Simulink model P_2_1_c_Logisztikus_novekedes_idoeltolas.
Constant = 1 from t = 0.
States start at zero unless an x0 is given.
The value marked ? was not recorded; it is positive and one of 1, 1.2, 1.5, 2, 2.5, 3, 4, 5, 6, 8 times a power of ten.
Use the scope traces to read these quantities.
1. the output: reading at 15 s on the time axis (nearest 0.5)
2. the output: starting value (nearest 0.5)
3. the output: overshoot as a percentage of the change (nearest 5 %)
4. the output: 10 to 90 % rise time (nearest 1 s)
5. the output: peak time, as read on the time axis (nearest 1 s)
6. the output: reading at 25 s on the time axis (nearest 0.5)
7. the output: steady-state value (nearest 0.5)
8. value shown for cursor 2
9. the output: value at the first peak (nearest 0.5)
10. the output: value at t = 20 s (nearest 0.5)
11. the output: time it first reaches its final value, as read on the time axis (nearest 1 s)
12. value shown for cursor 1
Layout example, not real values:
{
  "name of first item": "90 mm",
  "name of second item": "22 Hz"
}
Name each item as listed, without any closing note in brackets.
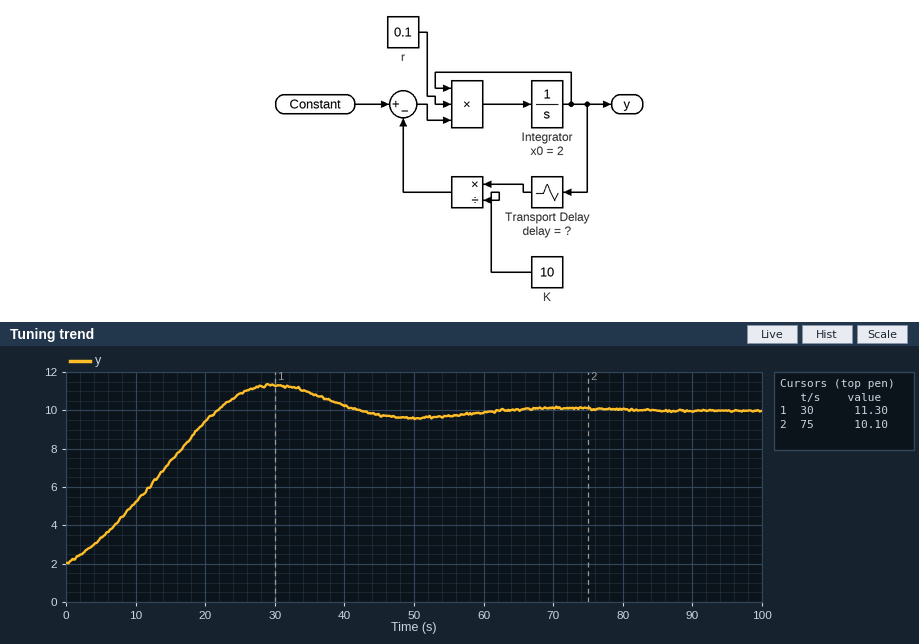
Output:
{
  "the output: reading at 15 s on the time axis": "7.5",
  "the output: starting value": "2.0",
  "the output: overshoot as a percentage of the change": "15 %",
  "the output: 10 to 90 % rise time": "16 s",
  "the output: peak time, as read on the time axis": "30 s",
  "the output: reading at 25 s on the time axis": "11.0",
  "the output: steady-state value": "10.0",
  "value shown for cursor 2": "10.10",
  "the output: value at the first peak": "11.5",
  "the output: value at t = 20 s": "9.5",
  "the output: time it first reaches its final value, as read on the time axis": "22 s",
  "value shown for cursor 1": "11.30"
}
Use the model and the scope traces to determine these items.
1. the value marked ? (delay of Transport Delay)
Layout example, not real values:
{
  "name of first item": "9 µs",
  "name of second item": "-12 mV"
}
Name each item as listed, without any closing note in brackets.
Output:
{
  "the value marked ?": "8"
}
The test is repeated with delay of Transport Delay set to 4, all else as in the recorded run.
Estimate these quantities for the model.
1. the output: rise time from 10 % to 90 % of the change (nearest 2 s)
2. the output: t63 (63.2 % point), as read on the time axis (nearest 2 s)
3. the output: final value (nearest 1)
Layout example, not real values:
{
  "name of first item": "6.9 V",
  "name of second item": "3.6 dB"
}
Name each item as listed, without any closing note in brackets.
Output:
{
  "the output: rise time from 10 % to 90 % of the change": "24 s",
  "the output: t63 (63.2 % point), as read on the time axis": "18 s",
  "the output: final value": "10"
}
